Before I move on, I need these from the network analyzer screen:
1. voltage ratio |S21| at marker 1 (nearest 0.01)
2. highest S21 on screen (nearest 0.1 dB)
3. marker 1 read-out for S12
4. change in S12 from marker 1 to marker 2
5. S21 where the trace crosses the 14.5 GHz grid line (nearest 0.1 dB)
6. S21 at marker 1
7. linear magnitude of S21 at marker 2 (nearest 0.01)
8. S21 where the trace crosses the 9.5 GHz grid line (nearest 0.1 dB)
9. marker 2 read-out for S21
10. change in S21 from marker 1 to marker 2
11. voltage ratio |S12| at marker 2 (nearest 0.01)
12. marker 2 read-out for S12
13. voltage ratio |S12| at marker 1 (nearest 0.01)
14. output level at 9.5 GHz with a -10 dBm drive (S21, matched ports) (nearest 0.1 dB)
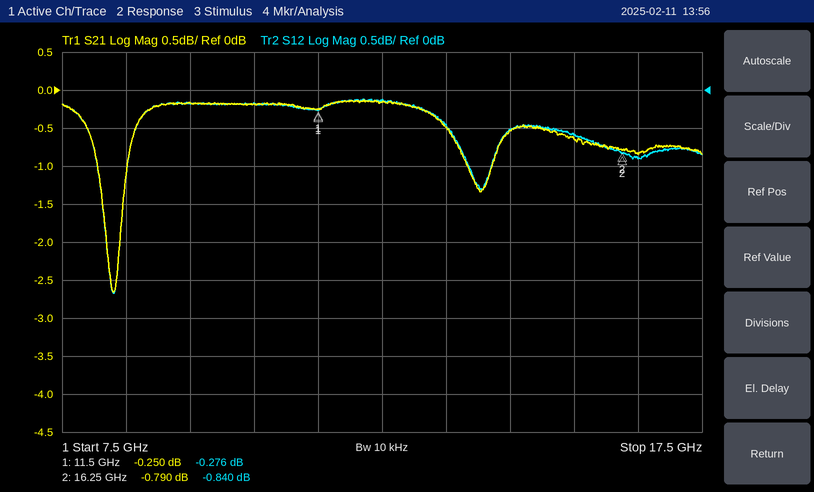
0.97
-0.1 dB
-0.276 dB
-0.564 dB
-0.5 dB
-0.250 dB
0.91
-0.2 dB
-0.790 dB
-0.540 dB
0.91
-0.840 dB
0.97
-10.2 dBm
